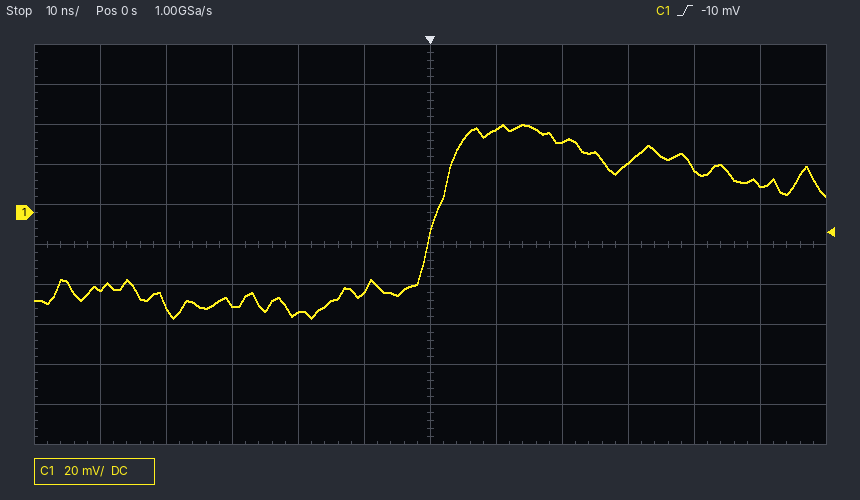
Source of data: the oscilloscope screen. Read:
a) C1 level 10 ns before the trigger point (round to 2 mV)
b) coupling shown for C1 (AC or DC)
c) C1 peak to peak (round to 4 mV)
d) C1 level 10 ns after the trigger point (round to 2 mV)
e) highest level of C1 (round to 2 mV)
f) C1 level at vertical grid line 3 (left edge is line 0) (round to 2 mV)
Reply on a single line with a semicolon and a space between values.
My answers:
-40 mV; DC; 96 mV; 42 mV; 44 mV; -46 mV
